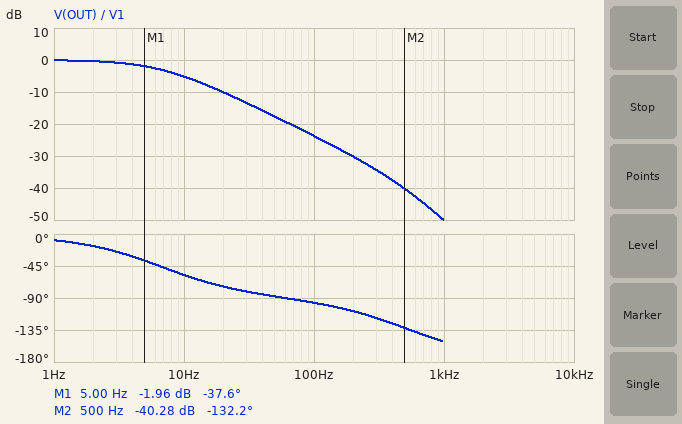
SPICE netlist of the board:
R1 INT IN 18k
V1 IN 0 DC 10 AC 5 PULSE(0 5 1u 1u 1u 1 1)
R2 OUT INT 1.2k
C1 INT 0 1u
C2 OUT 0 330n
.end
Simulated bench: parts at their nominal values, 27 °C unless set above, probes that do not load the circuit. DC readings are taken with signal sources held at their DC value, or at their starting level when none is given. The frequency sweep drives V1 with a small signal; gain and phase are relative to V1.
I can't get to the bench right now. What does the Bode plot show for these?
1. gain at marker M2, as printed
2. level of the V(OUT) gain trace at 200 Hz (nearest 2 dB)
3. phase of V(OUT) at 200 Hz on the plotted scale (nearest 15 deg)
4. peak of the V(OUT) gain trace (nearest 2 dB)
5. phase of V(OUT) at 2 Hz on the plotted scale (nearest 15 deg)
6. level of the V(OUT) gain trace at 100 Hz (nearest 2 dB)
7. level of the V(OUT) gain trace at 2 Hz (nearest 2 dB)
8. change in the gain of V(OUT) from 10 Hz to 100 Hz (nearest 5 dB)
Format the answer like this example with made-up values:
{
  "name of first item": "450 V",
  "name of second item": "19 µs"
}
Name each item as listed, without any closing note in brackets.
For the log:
{
  "gain at marker M2, as printed": "-40.28 dB",
  "level of the V(OUT) gain trace at 200 Hz": "-30 dB",
  "phase of V(OUT) at 200 Hz on the plotted scale": "-105 deg",
  "peak of the V(OUT) gain trace": "0 dB",
  "phase of V(OUT) at 2 Hz on the plotted scale": "-15 deg",
  "level of the V(OUT) gain trace at 100 Hz": "-24 dB",
  "level of the V(OUT) gain trace at 2 Hz": "0 dB",
  "change in the gain of V(OUT) from 10 Hz to 100 Hz": "-20 dB"
}
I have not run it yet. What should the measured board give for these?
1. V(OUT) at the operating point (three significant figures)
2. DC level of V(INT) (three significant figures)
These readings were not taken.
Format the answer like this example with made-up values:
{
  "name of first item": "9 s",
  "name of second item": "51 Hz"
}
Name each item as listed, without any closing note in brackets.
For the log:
{
  "V(OUT) at the operating point": "10.0 V",
  "DC level of V(INT)": "10.0 V"
}
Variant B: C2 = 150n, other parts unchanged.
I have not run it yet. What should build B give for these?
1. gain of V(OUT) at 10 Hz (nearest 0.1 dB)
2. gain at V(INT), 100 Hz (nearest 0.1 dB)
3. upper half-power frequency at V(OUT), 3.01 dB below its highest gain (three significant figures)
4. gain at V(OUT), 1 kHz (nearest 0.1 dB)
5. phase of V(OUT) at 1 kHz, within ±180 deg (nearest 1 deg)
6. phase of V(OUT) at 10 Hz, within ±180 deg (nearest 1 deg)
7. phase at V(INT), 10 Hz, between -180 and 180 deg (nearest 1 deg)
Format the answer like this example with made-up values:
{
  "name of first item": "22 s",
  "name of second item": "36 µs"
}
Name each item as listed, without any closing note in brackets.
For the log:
{
  "gain of V(OUT) at 10 Hz": "-4.3 dB",
  "gain at V(INT), 100 Hz": "-22.3 dB",
  "upper half-power frequency at V(OUT), 3.01 dB below its highest gain": "7.68 Hz",
  "gain at V(OUT), 1 kHz": "-45.2 dB",
  "phase of V(OUT) at 1 kHz, within ±180 deg": "-134 deg",
  "phase of V(OUT) at 10 Hz, within ±180 deg": "-53 deg",
  "phase at V(INT), 10 Hz, between -180 and 180 deg": "-52 deg"
}
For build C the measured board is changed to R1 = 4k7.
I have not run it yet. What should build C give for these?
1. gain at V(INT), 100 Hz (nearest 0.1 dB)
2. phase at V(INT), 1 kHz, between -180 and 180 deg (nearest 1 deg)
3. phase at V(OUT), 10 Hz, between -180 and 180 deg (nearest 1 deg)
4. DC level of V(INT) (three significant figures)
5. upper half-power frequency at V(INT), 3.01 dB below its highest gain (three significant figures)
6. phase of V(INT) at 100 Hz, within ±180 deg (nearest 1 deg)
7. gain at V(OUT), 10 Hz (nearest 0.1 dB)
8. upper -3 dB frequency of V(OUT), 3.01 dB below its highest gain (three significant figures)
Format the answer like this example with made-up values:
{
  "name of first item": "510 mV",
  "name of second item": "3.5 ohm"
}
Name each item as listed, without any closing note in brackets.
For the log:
{
  "gain at V(INT), 100 Hz": "-12.2 dB",
  "phase at V(INT), 1 kHz, between -180 and 180 deg": "-82 deg",
  "phase at V(OUT), 10 Hz, between -180 and 180 deg": "-23 deg",
  "DC level of V(INT)": "10.0 V",
  "upper half-power frequency at V(INT), 3.01 dB below its highest gain": "25.1 Hz",
  "phase of V(INT) at 100 Hz, within ±180 deg": "-72 deg",
  "gain at V(OUT), 10 Hz": "-0.6 dB",
  "upper -3 dB frequency of V(OUT), 3.01 dB below its highest gain": "25.0 Hz"
}
